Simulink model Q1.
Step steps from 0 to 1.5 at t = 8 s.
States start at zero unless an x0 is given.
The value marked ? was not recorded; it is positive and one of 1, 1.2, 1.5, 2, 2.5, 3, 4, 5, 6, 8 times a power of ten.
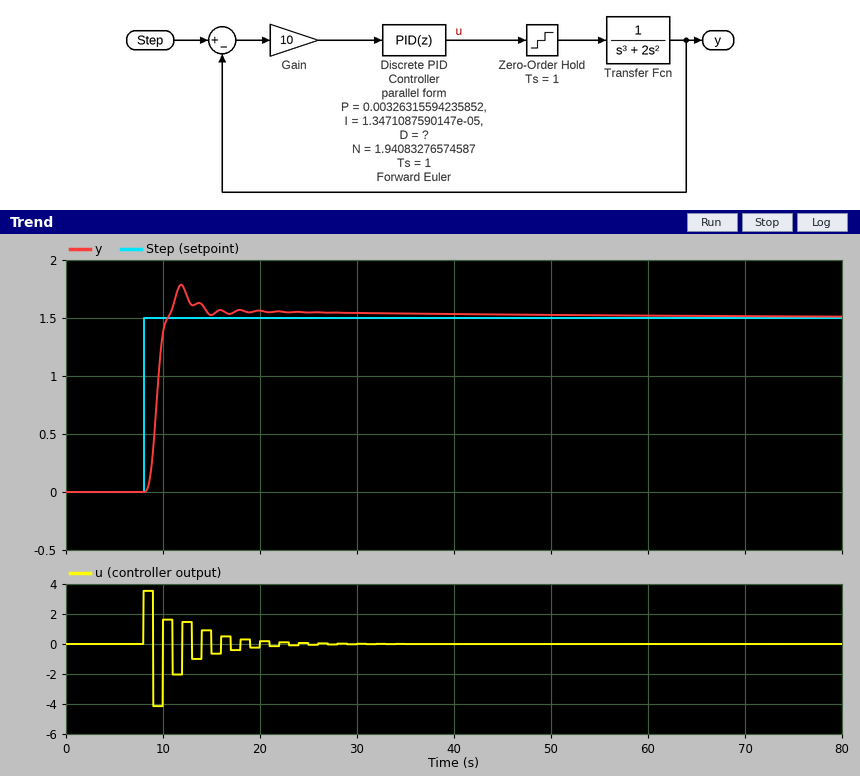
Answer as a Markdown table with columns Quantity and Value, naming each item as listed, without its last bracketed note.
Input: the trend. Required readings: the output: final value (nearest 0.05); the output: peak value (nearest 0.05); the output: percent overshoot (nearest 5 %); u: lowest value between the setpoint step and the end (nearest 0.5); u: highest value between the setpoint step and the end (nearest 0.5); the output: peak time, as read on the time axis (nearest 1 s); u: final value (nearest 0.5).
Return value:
| Quantity | Value |
|---|---|
| the output: final value | 1.50 |
| the output: peak value | 1.80 |
| the output: percent overshoot | 20 % |
| u: lowest value between the setpoint step and the end | -4.0 |
| u: highest value between the setpoint step and the end | 3.5 |
| the output: peak time, as read on the time axis | 12 s |
| u: final value | 0.0 |
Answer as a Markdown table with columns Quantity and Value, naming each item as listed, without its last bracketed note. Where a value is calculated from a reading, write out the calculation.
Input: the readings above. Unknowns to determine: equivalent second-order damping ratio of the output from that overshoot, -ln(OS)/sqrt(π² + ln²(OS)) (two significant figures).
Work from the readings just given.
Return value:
| Quantity | Value |
|---|---|
| equivalent second-order damping ratio of the output from that overshoot, -ln(OS)/sqrt(π² + ln²(OS)) | ln(0.2) = -1.609; 1.609 / sqrt(9.870 + 2.590) = 0.46 |
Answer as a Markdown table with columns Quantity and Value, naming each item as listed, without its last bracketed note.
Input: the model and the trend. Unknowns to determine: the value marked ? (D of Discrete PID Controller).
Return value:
| Quantity | Value |
|---|---|
| the value marked ? | 0.12 |
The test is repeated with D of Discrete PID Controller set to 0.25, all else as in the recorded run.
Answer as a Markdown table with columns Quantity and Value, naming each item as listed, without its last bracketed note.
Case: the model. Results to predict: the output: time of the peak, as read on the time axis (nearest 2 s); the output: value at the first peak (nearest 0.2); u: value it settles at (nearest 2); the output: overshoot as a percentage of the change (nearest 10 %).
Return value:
| Quantity | Value |
|---|---|
| the output: time of the peak, as read on the time axis | 10 s |
| the output: value at the first peak | 2.6 |
| u: value it settles at | 0 |
| the output: overshoot as a percentage of the change | 80 % |
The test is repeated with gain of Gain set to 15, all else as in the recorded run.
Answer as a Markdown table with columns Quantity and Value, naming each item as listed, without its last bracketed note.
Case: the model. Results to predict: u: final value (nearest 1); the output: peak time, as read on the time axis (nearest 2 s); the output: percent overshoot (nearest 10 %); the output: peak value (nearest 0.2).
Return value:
| Quantity | Value |
|---|---|
| u: final value | 0 |
| the output: peak time, as read on the time axis | 10 s |
| the output: percent overshoot | 40 % |
| the output: peak value | 2.0 |
